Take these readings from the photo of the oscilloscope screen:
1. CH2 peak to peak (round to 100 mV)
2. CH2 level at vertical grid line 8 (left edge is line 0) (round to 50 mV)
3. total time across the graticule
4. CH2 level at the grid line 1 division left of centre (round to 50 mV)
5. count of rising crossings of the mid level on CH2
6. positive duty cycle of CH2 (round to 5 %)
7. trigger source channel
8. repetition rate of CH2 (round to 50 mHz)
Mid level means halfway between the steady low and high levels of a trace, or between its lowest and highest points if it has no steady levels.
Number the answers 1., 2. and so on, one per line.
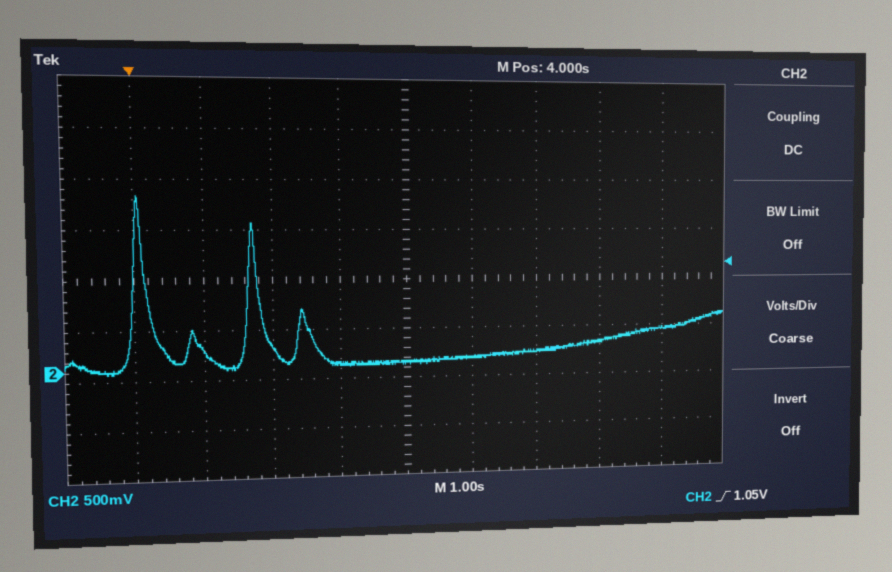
1. 1.80 V
2. 250 mV
3. 10 s
4. 50 mV
5. 2
6. 10 %
7. CH2
8. 600 mHz
